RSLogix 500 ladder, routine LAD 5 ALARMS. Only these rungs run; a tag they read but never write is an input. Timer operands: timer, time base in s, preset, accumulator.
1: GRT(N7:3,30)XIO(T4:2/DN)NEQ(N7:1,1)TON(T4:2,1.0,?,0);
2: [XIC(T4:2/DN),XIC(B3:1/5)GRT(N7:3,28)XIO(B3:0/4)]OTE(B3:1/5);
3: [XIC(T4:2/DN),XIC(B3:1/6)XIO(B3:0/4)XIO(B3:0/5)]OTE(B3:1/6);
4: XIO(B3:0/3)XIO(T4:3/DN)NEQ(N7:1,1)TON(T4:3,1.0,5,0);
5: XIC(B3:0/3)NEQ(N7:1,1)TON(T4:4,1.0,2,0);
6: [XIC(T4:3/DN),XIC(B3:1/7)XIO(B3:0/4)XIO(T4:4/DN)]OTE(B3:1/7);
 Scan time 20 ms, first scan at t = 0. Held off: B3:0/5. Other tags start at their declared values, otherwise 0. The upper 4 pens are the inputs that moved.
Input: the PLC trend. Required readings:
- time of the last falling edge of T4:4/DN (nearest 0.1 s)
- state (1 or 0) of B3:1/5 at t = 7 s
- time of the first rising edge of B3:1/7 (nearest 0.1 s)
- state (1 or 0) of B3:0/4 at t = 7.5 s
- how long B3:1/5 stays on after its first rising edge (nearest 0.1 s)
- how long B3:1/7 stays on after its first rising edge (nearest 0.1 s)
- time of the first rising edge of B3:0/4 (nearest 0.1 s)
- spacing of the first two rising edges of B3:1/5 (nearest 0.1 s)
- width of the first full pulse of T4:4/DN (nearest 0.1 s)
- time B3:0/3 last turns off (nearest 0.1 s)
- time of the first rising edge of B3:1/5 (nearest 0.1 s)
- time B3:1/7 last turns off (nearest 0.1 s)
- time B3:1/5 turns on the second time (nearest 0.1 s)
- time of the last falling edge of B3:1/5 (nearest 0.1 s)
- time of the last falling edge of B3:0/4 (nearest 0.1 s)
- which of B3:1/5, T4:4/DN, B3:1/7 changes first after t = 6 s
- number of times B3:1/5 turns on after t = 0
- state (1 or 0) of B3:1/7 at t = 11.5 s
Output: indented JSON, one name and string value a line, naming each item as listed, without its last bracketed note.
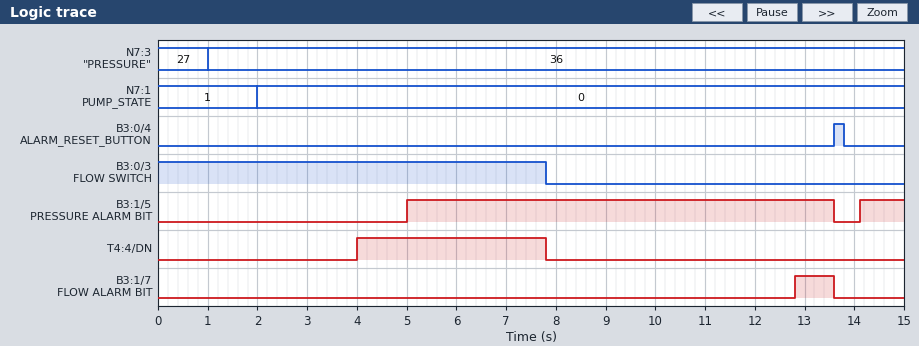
{
  "time of the last falling edge of T4:4/DN": "7.8 s",
  "state (1 or 0) of B3:1/5 at t = 7 s": "1",
  "time of the first rising edge of B3:1/7": "12.8 s",
  "state (1 or 0) of B3:0/4 at t = 7.5 s": "0",
  "how long B3:1/5 stays on after its first rising edge": "8.6 s",
  "how long B3:1/7 stays on after its first rising edge": "0.8 s",
  "time of the first rising edge of B3:0/4": "13.6 s",
  "spacing of the first two rising edges of B3:1/5": "9.1 s",
  "width of the first full pulse of T4:4/DN": "3.8 s",
  "time B3:0/3 last turns off": "7.8 s",
  "time of the first rising edge of B3:1/5": "5.0 s",
  "time B3:1/7 last turns off": "13.6 s",
  "time B3:1/5 turns on the second time": "14.1 s",
  "time of the last falling edge of B3:1/5": "13.6 s",
  "time of the last falling edge of B3:0/4": "13.8 s",
  "which of B3:1/5, T4:4/DN, B3:1/7 changes first after t = 6 s": "T4:4/DN",
  "number of times B3:1/5 turns on after t = 0": "2",
  "state (1 or 0) of B3:1/7 at t = 11.5 s": "0"
}
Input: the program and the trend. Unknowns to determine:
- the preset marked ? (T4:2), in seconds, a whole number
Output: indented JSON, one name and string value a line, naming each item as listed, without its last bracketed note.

{
  "the preset marked ? (T4:2), in seconds, a whole number": "3 s"
}
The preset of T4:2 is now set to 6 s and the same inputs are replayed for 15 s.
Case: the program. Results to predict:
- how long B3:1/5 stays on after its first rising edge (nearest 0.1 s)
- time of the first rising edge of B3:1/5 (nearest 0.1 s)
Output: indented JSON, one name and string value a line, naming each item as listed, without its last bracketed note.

{
  "how long B3:1/5 stays on after its first rising edge": "5.6 s",
  "time of the first rising edge of B3:1/5": "8.0 s"
}
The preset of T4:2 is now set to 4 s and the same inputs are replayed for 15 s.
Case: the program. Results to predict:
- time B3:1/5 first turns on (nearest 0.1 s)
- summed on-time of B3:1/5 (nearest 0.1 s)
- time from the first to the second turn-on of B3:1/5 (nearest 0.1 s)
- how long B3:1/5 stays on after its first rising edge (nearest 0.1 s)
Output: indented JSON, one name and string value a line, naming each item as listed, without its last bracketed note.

{
  "time B3:1/5 first turns on": "6.0 s",
  "summed on-time of B3:1/5": "8.5 s",
  "time from the first to the second turn-on of B3:1/5": "8.1 s",
  "how long B3:1/5 stays on after its first rising edge": "7.6 s"
}
